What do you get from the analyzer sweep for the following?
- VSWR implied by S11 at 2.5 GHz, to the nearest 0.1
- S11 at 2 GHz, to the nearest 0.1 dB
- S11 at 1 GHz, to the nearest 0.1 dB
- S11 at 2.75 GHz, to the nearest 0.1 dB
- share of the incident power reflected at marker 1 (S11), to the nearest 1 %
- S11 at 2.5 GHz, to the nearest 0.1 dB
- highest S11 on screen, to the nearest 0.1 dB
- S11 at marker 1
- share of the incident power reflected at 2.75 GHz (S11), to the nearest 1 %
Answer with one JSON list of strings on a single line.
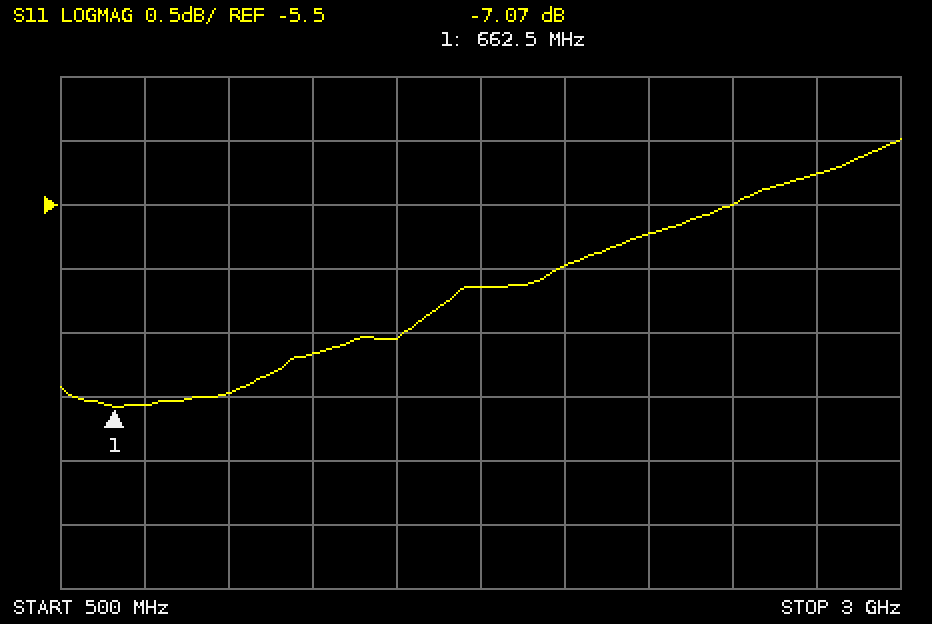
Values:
["3.3", "-6.0 dB", "-7.0 dB", "-5.3 dB", "20 %", "-5.5 dB", "-5.0 dB", "-7.07 dB", "30 %"]
